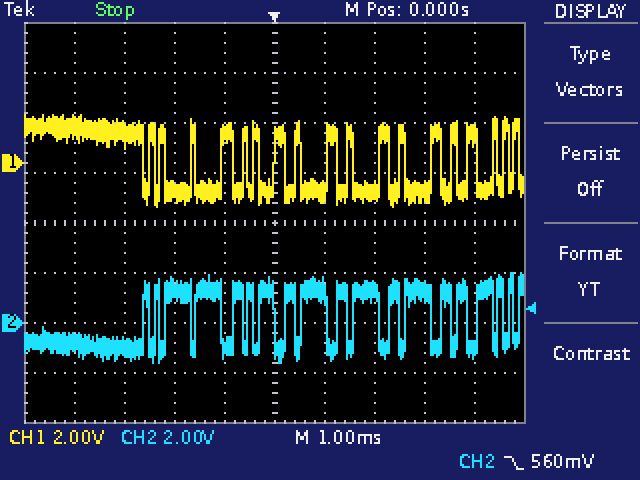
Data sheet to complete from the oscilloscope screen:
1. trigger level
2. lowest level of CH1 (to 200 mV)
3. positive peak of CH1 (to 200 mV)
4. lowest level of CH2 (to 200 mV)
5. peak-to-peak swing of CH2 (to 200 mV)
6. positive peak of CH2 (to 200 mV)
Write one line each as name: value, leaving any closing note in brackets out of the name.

trigger level: 560 mV
lowest level of CH1: -1.8 V
positive peak of CH1: 2.0 V
lowest level of CH2: -1.6 V
peak-to-peak swing of CH2: 3.6 V
positive peak of CH2: 2.0 V
